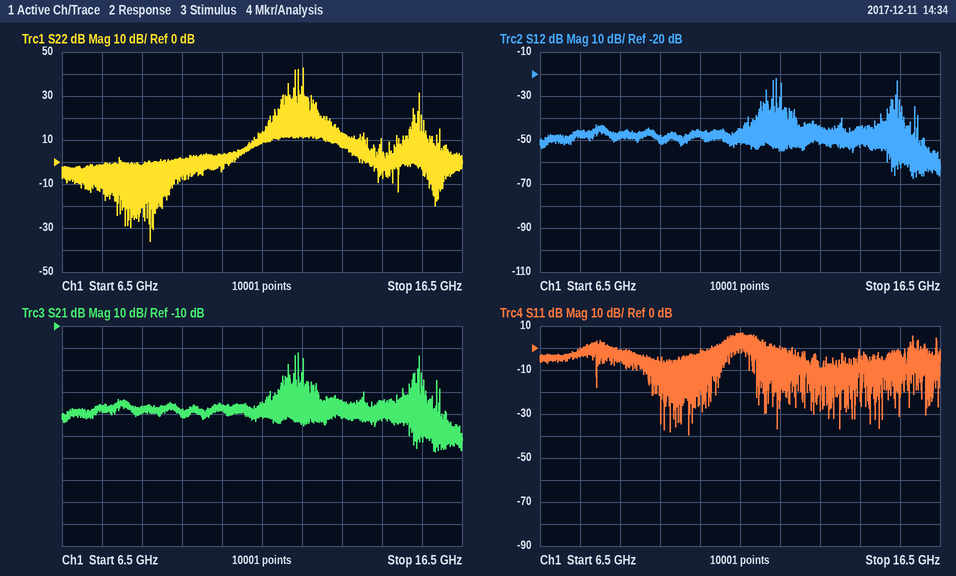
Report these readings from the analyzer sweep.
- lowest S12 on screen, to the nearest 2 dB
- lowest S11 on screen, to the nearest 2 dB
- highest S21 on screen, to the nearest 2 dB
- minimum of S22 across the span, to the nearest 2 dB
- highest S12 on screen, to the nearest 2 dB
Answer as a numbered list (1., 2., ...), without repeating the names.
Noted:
1. -68 dB
2. -40 dB
3. -22 dB
4. -36 dB
5. -22 dB
